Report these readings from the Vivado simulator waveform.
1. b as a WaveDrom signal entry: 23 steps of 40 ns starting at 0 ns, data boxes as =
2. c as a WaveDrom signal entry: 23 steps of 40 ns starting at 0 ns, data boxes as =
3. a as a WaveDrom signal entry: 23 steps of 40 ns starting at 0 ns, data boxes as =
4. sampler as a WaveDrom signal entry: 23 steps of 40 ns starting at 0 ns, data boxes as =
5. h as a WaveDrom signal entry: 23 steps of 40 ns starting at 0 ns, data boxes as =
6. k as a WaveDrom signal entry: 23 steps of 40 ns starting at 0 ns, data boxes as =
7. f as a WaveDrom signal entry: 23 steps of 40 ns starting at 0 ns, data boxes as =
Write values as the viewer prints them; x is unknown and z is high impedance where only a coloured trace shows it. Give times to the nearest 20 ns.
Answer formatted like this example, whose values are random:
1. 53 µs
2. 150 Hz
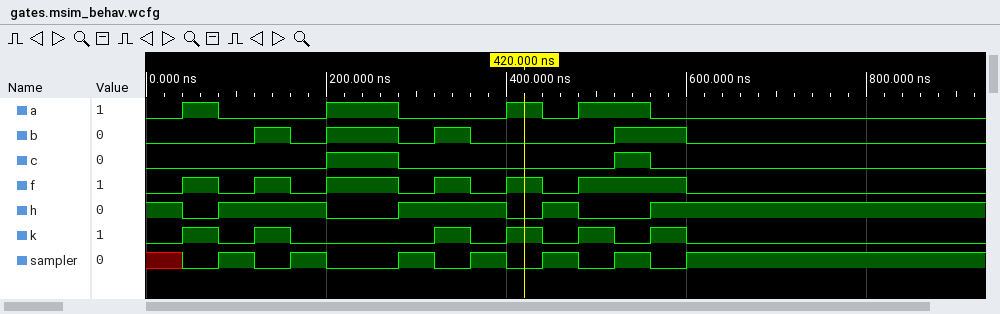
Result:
1. {name: 'b', wave: '0..101.010...1.0.......'}
2. {name: 'c', wave: '0....1.0.....10........'}
3. {name: 'a', wave: '010..1.0..101.0........'}
4. {name: 'sampler', wave: 'x01010.101010101.......'}
5. {name: 'h', wave: '101..0.1..010.1........'}
6. {name: 'k', wave: '01010...10101010.......'}
7. {name: 'f', wave: '010101.010101..0.......'}
